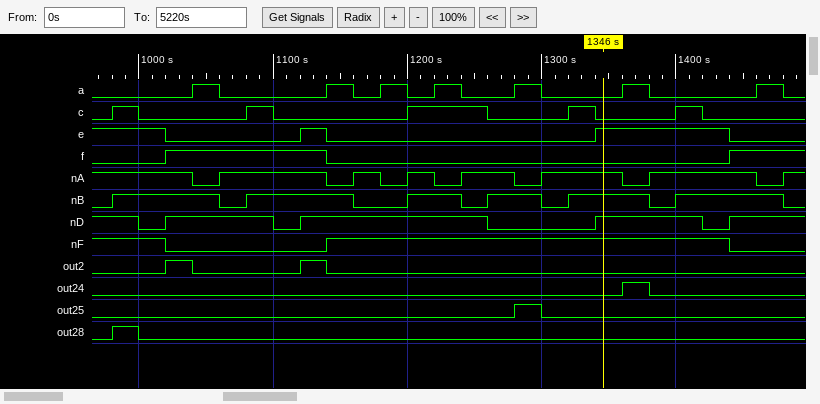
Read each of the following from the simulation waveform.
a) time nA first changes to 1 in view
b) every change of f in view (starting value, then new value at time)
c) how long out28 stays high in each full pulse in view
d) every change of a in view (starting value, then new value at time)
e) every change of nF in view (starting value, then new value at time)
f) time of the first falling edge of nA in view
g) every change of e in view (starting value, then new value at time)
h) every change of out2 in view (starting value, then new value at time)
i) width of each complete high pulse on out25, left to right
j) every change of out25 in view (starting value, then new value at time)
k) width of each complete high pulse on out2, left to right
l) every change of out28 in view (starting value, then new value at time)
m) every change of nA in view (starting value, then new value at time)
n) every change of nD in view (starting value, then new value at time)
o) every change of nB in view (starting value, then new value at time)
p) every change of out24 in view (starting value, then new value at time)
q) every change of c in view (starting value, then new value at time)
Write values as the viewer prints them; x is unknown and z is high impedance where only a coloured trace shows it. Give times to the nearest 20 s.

1060 s
0, 1 at 1020 s, 0 at 1140 s, 1 at 1440 s
20 s
0, 1 at 1040 s, 0 at 1060 s, 1 at 1140 s, 0 at 1160 s, 1 at 1180 s, 0 at 1200 s, 1 at 1220 s, 0 at 1240 s, 1 at 1280 s, 0 at 1300 s, 1 at 1360 s, 0 at 1380 s, 1 at 1460 s, 0 at 1480 s
1, 0 at 1020 s, 1 at 1140 s, 0 at 1440 s
1040 s
1, 0 at 1020 s, 1 at 1120 s, 0 at 1140 s, 1 at 1340 s, 0 at 1440 s
0, 1 at 1020 s, 0 at 1040 s, 1 at 1120 s, 0 at 1140 s
20 s
0, 1 at 1280 s, 0 at 1300 s
20 s, 20 s
0, 1 at 980 s, 0 at 1000 s
1, 0 at 1040 s, 1 at 1060 s, 0 at 1140 s, 1 at 1160 s, 0 at 1180 s, 1 at 1200 s, 0 at 1220 s, 1 at 1240 s, 0 at 1280 s, 1 at 1300 s, 0 at 1360 s, 1 at 1380 s, 0 at 1460 s, 1 at 1480 s
1, 0 at 1000 s, 1 at 1020 s, 0 at 1100 s, 1 at 1120 s, 0 at 1260 s, 1 at 1340 s, 0 at 1420 s, 1 at 1440 s
0, 1 at 980 s, 0 at 1060 s, 1 at 1080 s, 0 at 1160 s, 1 at 1200 s, 0 at 1240 s, 1 at 1260 s, 0 at 1300 s, 1 at 1320 s, 0 at 1380 s, 1 at 1400 s, 0 at 1480 s
0, 1 at 1360 s, 0 at 1380 s
0, 1 at 980 s, 0 at 1000 s, 1 at 1080 s, 0 at 1100 s, 1 at 1200 s, 0 at 1260 s, 1 at 1320 s, 0 at 1340 s, 1 at 1400 s, 0 at 1420 s
